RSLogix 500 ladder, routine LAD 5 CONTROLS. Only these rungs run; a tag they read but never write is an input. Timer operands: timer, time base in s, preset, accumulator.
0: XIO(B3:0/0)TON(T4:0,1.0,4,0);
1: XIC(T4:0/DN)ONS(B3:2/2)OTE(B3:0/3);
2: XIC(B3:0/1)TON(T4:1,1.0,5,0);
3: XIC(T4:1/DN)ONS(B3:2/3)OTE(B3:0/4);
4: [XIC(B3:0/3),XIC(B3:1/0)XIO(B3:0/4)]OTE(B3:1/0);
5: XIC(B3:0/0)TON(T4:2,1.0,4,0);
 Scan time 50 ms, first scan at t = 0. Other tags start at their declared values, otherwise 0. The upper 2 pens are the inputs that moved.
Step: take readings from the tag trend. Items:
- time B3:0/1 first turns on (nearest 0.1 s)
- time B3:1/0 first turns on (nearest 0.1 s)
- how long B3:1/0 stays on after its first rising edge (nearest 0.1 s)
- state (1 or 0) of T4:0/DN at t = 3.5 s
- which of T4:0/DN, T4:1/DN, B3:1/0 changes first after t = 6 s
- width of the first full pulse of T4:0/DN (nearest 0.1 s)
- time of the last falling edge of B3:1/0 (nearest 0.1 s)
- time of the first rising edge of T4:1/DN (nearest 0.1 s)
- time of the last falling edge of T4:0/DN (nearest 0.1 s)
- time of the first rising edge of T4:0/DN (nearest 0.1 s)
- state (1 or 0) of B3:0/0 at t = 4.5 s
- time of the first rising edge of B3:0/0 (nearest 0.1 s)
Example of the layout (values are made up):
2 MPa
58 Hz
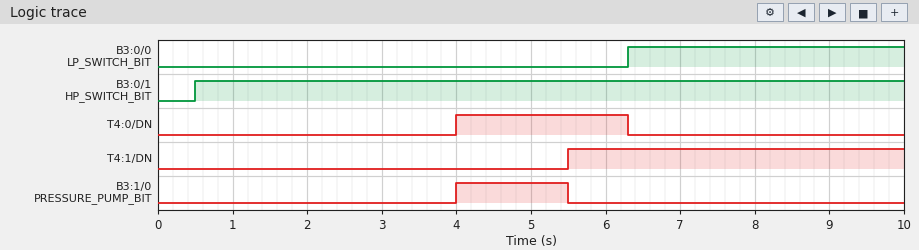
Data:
0.5 s
4.0 s
1.5 s
0
T4:0/DN
2.3 s
5.5 s
5.5 s
6.3 s
4.0 s
0
6.3 s
